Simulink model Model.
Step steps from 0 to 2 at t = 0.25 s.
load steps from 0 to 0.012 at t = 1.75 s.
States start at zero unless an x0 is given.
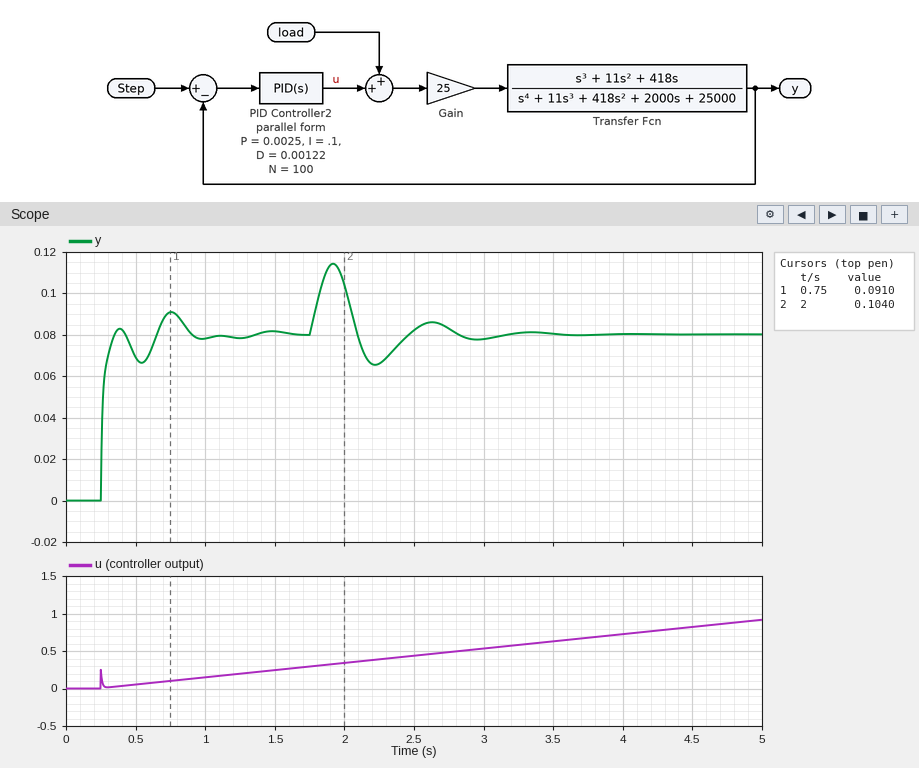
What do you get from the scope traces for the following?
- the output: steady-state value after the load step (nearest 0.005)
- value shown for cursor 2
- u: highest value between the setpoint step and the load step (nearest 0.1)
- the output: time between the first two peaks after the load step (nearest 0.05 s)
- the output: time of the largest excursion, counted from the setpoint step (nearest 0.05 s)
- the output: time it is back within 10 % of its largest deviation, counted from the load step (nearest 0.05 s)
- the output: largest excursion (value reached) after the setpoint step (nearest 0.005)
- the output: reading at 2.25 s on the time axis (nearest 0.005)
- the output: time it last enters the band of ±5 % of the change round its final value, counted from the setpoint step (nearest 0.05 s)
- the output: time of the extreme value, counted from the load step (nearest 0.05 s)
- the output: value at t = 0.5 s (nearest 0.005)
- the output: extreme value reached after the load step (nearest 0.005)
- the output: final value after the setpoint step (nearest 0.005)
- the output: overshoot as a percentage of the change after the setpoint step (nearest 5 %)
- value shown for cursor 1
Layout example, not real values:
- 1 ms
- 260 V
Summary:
- 0.080
- 0.1040
- 0.3
- 0.70 s
- 0.50 s
- 1.00 s
- 0.090
- 0.065
- 0.60 s
- 0.15 s
- 0.070
- 0.115
- 0.080
- 15 %
- 0.0910
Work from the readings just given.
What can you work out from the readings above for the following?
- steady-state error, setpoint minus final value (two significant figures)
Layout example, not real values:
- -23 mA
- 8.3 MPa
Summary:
- 1.9
